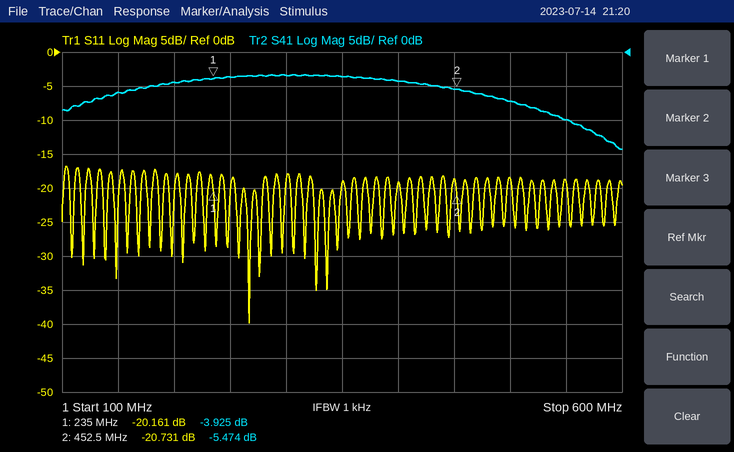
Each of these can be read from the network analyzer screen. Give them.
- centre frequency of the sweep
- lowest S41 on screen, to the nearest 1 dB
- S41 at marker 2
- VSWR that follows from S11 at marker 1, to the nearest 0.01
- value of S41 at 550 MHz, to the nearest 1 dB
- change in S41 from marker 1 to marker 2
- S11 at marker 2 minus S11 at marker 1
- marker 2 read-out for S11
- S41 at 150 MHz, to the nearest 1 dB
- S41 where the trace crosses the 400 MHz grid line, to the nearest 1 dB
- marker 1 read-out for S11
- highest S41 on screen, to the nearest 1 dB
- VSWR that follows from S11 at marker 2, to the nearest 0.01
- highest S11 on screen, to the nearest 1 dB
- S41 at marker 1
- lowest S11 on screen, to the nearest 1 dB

350 MHz
-14 dB
-5.474 dB
1.22
-10 dB
-1.549 dB
-0.570 dB
-20.731 dB
-6 dB
-4 dB
-20.161 dB
-3 dB
1.20
-17 dB
-3.925 dB
-40 dB
